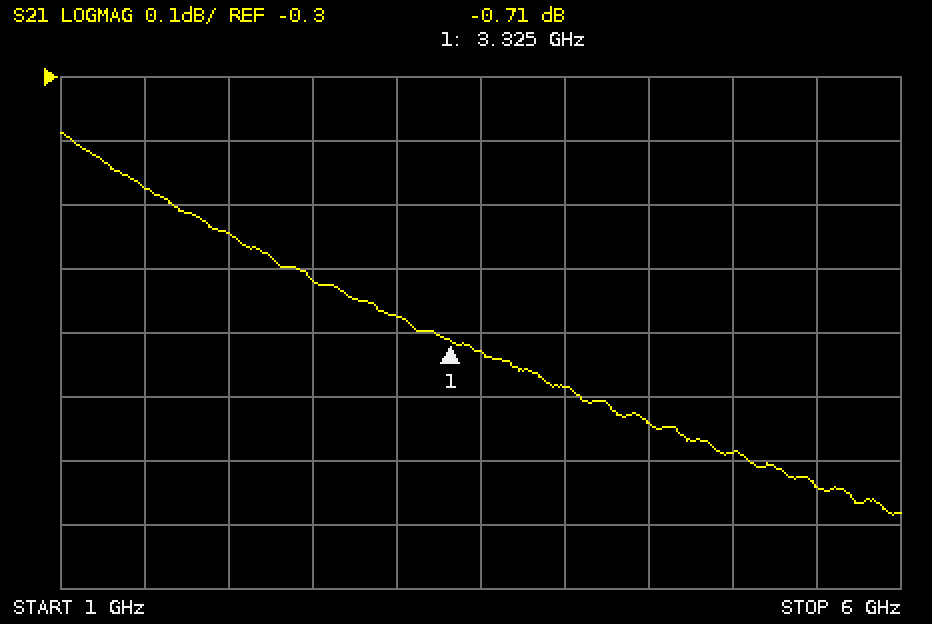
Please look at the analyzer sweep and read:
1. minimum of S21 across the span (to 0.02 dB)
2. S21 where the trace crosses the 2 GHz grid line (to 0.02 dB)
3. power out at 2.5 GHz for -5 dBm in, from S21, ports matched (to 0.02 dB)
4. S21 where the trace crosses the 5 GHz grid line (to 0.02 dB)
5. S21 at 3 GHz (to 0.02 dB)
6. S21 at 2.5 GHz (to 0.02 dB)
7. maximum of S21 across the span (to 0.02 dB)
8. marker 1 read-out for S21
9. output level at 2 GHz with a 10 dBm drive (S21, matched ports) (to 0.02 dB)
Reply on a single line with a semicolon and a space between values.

-0.98 dB; -0.54 dB; -5.62 dBm; -0.88 dB; -0.68 dB; -0.62 dB; -0.38 dB; -0.71 dB; 9.46 dBm
